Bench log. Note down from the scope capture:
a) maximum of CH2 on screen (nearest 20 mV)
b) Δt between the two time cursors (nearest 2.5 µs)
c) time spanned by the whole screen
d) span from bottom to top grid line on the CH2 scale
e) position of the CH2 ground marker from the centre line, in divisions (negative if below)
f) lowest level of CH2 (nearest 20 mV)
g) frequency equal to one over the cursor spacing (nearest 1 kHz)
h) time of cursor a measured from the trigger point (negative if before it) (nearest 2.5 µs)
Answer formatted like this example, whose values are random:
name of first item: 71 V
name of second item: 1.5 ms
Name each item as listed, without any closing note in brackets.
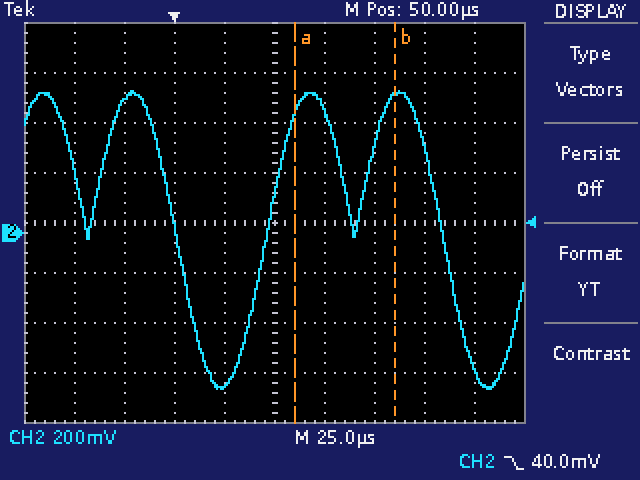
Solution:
maximum of CH2 on screen: 560 mV
Δt between the two time cursors: 50.0 µs
time spanned by the whole screen: 250 µs
span from bottom to top grid line on the CH2 scale: 1.6 V
position of the CH2 ground marker from the centre line, in divisions: -0.2 div
lowest level of CH2: -620 mV
frequency equal to one over the cursor spacing: 20 kHz
time of cursor a measured from the trigger point (negative if before it): +60.0 µs
